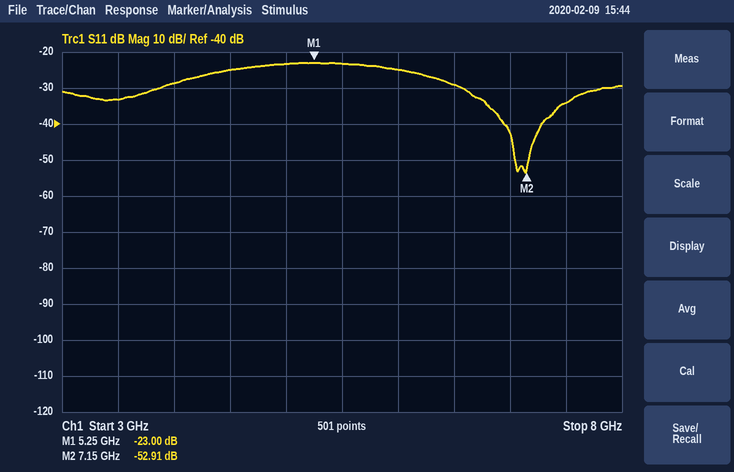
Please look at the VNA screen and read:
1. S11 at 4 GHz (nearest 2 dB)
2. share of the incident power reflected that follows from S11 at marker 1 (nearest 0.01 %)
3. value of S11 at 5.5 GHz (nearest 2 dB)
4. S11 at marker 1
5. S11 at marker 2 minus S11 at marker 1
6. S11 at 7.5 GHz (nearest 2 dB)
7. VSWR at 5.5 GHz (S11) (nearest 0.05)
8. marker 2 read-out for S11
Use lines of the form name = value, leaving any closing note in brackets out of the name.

S11 at 4 GHz = -28 dB
share of the incident power reflected that follows from S11 at marker 1 = 0.50 %
value of S11 at 5.5 GHz = -24 dB
S11 at marker 1 = -23.00 dB
S11 at marker 2 minus S11 at marker 1 = -29.91 dB
S11 at 7.5 GHz = -34 dB
VSWR at 5.5 GHz (S11) = 1.15
marker 2 read-out for S11 = -52.91 dB
